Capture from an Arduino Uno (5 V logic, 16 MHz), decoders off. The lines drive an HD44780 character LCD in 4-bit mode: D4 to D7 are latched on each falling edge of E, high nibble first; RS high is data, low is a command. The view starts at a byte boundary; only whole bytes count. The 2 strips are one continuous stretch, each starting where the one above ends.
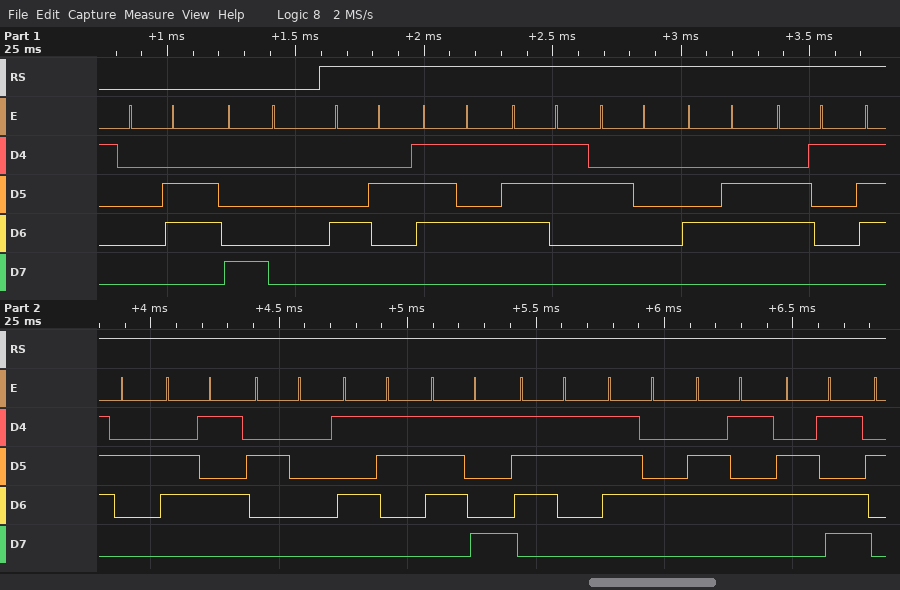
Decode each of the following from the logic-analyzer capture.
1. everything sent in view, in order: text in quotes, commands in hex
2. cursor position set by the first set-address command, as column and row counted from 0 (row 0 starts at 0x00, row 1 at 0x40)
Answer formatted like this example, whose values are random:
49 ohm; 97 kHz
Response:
0x06 0x80 "Bus Fare System"; column 0, row 0
